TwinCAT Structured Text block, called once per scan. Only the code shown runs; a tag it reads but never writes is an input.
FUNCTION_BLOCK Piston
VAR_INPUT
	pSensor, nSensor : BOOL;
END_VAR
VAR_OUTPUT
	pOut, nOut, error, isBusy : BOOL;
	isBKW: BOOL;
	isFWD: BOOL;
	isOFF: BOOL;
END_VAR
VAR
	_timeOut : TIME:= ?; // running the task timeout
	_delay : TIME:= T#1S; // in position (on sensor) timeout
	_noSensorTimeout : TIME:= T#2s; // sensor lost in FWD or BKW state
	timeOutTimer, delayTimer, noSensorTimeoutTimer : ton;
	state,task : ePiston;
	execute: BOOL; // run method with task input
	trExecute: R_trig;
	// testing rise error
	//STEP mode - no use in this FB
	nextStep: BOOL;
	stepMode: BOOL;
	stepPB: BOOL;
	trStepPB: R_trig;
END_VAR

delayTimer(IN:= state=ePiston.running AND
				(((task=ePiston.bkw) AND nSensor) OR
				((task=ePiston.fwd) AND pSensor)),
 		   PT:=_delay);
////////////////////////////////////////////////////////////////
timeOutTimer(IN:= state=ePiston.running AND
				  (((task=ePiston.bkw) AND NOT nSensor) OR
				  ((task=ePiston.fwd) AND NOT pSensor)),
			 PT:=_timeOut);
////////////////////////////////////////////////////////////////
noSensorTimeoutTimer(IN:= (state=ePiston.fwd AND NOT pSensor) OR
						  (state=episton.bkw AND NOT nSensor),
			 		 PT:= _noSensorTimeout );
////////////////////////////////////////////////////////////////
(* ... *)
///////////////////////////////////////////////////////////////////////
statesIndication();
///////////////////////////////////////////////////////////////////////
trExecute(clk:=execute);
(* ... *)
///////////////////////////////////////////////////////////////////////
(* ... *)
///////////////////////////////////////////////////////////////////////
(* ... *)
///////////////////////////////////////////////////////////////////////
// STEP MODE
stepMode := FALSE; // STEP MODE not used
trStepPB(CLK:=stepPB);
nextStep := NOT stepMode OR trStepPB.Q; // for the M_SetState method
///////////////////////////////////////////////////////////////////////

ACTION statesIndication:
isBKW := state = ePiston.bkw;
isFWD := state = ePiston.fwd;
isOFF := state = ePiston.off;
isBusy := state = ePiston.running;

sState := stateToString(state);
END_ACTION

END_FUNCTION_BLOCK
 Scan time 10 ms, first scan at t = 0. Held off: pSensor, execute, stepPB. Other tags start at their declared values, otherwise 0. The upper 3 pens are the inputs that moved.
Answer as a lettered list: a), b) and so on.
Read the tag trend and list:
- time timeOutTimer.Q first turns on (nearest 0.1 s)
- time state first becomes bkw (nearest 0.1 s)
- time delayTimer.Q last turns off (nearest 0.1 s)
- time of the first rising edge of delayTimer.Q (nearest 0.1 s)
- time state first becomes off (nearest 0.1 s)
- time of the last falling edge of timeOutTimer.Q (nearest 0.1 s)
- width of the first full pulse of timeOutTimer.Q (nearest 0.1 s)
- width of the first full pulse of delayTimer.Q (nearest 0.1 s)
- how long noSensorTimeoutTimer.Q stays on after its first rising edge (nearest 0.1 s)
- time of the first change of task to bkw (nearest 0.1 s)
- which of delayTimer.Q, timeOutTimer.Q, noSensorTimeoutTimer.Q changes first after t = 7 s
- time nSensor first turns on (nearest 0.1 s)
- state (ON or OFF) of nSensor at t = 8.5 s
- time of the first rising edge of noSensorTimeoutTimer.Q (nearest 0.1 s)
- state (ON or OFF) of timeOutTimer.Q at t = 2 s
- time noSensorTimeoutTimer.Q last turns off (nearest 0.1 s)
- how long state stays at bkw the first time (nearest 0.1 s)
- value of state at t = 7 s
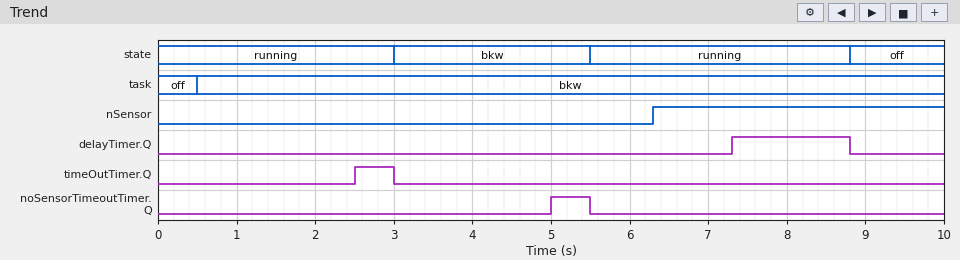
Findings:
a) 2.5 s
b) 3.0 s
c) 8.8 s
d) 7.3 s
e) 8.8 s
f) 3.0 s
g) 0.5 s
h) 1.5 s
i) 0.5 s
j) 0.5 s
k) delayTimer.Q
l) 6.3 s
m) ON
n) 5.0 s
o) OFF
p) 5.5 s
q) 2.5 s
r) running
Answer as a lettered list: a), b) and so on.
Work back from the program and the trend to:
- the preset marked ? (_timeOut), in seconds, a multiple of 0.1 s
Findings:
a) 2.0 s
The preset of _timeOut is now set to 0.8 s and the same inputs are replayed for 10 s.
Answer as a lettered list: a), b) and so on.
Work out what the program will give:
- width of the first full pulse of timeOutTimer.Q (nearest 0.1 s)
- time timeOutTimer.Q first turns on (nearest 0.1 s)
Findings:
a) 1.7 s
b) 1.3 s
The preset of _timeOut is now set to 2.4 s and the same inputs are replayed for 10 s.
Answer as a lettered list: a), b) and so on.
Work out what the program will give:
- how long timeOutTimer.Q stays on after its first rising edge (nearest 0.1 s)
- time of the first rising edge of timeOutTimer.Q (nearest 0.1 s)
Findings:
a) 0.1 s
b) 2.9 s
